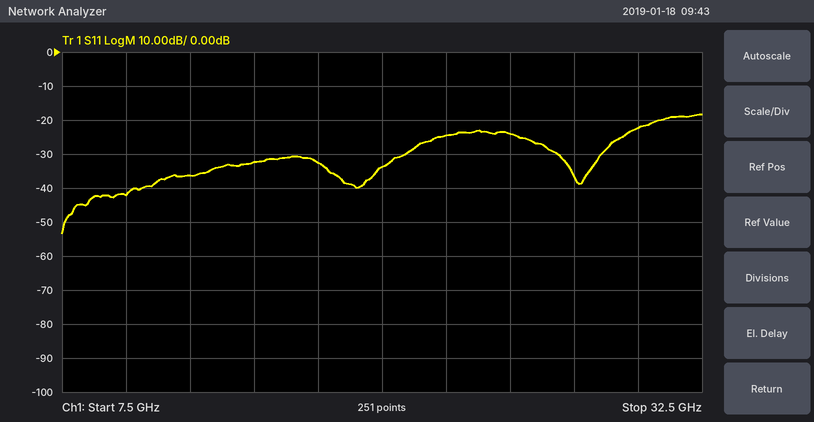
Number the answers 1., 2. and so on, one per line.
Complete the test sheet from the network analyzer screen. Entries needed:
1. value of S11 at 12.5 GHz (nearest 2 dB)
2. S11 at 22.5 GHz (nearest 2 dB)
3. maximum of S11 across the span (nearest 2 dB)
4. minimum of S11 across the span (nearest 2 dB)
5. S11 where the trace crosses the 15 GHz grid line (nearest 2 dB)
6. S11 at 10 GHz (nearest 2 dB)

1. -36 dB
2. -24 dB
3. -18 dB
4. -54 dB
5. -32 dB
6. -42 dB
